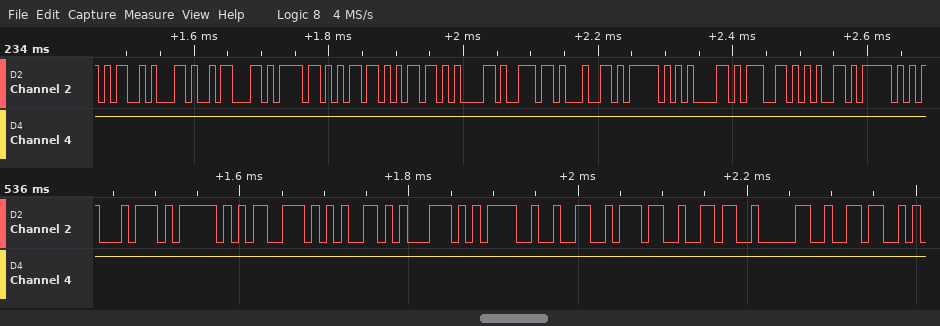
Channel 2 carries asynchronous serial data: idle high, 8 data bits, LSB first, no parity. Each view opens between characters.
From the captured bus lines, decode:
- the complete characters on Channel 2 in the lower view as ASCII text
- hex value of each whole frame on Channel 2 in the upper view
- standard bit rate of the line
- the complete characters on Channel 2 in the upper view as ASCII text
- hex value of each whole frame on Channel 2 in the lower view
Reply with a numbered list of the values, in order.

1. "t_seq=27606"
2. 4D, 2C, 63, 6F, 6D, 6D, 61, 6E, 64, 5F, 61, 67, 65, 5F
3. 115200 baud
4. "M,command_age_"
5. 74, 5F, 73, 65, 71, 3D, 32, 37, 36, 30, 36
